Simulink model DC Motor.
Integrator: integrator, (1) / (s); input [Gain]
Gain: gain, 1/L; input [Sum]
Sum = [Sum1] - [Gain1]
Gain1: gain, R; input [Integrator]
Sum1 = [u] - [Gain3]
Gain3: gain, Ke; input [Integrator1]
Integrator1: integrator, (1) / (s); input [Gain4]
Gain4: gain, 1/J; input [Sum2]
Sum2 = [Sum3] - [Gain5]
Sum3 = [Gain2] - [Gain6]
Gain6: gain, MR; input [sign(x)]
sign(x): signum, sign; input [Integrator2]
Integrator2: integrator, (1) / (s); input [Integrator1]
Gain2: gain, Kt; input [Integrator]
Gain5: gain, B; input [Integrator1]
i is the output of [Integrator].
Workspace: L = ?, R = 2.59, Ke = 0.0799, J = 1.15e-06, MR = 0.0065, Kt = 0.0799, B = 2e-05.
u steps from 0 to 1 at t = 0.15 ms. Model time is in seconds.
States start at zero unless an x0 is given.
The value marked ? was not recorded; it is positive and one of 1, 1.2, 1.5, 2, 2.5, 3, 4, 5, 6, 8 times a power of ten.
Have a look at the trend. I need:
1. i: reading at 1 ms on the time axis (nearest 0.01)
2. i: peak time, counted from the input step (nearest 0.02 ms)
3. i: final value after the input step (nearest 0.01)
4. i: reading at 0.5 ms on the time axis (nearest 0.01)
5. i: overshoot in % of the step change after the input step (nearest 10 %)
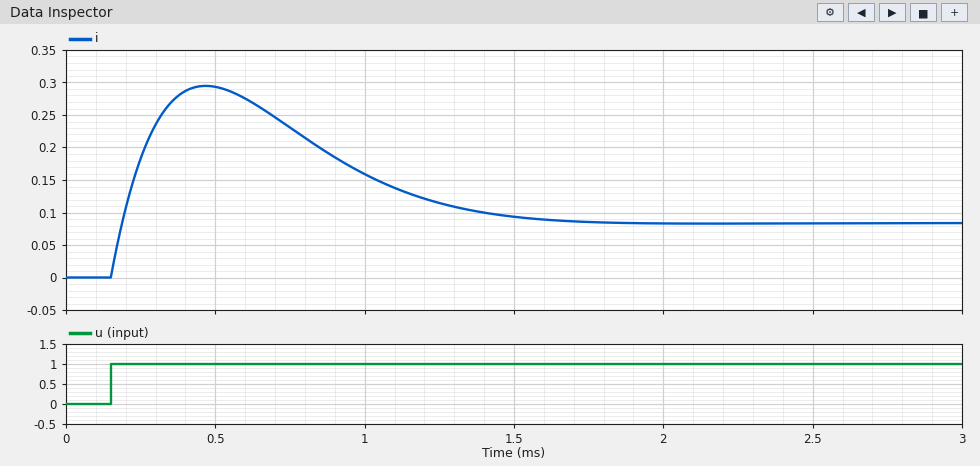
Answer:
0.16
0.32 ms
0.08
0.29
250 %
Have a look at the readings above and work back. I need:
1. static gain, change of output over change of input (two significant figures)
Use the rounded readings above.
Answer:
0.080
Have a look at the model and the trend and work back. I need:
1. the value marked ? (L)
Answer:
0.0004
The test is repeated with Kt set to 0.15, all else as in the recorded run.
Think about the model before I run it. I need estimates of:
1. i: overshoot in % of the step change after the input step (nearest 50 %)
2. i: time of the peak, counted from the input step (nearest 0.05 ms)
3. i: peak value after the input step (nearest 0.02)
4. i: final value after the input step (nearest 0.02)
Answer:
450 %
0.25 ms
0.26
0.04
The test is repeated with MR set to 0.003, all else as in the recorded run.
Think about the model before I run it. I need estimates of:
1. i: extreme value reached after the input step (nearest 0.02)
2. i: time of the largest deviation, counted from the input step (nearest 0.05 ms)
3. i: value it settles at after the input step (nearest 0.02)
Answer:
0.28
0.30 ms
0.04
